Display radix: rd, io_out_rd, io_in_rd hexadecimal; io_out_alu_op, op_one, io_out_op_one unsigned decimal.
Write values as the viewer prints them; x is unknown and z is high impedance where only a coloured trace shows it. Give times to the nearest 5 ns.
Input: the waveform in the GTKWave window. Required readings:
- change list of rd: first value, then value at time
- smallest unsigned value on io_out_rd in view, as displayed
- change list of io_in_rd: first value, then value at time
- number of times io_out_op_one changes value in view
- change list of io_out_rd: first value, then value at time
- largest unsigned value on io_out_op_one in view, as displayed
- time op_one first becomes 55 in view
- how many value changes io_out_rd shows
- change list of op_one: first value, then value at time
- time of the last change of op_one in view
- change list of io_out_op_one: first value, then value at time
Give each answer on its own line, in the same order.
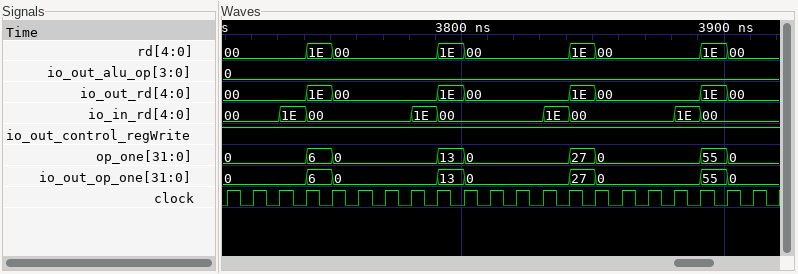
00, 1E at 3740 ns, 00 at 3750 ns, 1E at 3790 ns, 00 at 3800 ns, 1E at 3840 ns, 00 at 3850 ns, 1E at 3890 ns, 00 at 3900 ns
00
00, 1E at 3730 ns, 00 at 3740 ns, 1E at 3780 ns, 00 at 3790 ns, 1E at 3830 ns, 00 at 3840 ns, 1E at 3880 ns, 00 at 3890 ns
8
00, 1E at 3740 ns, 00 at 3750 ns, 1E at 3790 ns, 00 at 3800 ns, 1E at 3840 ns, 00 at 3850 ns, 1E at 3890 ns, 00 at 3900 ns
55
3890 ns
8
0, 6 at 3740 ns, 0 at 3750 ns, 13 at 3790 ns, 0 at 3800 ns, 27 at 3840 ns, 0 at 3850 ns, 55 at 3890 ns, 0 at 3900 ns
3900 ns
0, 6 at 3740 ns, 0 at 3750 ns, 13 at 3790 ns, 0 at 3800 ns, 27 at 3840 ns, 0 at 3850 ns, 55 at 3890 ns, 0 at 3900 ns
